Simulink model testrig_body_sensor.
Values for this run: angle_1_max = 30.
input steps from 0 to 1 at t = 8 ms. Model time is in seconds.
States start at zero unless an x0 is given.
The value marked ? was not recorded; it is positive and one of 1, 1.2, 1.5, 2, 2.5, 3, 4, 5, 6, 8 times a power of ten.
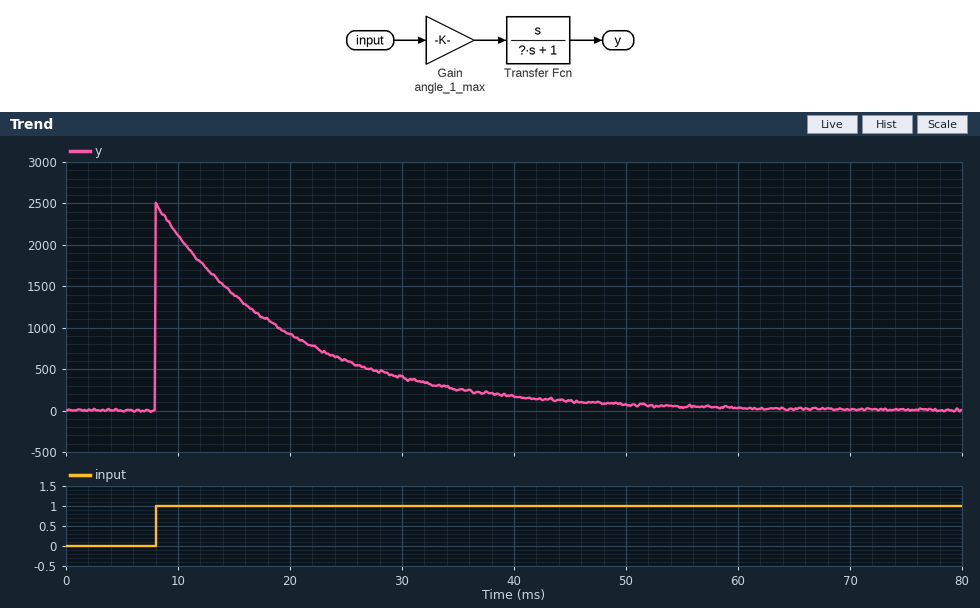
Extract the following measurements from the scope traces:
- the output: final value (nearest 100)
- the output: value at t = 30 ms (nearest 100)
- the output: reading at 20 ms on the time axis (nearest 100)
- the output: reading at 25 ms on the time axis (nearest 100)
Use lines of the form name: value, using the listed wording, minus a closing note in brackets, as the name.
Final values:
the output: final value: 0
the output: value at t = 30 ms: 400
the output: reading at 20 ms on the time axis: 900
the output: reading at 25 ms on the time axis: 600
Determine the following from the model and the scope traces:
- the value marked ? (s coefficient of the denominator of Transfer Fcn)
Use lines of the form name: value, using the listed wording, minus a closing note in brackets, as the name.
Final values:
the value marked ?: 0.012
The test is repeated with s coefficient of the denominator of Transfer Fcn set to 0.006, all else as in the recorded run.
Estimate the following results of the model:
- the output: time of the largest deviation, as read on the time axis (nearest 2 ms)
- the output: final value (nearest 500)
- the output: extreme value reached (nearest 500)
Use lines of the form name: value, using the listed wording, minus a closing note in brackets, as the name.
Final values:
the output: time of the largest deviation, as read on the time axis: 8 ms
the output: final value: 0
the output: extreme value reached: 5000
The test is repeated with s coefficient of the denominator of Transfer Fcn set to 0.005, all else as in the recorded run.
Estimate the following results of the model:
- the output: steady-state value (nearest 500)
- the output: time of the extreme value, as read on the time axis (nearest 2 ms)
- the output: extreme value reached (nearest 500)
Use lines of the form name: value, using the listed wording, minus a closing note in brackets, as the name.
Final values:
the output: steady-state value: 0
the output: time of the extreme value, as read on the time axis: 8 ms
the output: extreme value reached: 6000
